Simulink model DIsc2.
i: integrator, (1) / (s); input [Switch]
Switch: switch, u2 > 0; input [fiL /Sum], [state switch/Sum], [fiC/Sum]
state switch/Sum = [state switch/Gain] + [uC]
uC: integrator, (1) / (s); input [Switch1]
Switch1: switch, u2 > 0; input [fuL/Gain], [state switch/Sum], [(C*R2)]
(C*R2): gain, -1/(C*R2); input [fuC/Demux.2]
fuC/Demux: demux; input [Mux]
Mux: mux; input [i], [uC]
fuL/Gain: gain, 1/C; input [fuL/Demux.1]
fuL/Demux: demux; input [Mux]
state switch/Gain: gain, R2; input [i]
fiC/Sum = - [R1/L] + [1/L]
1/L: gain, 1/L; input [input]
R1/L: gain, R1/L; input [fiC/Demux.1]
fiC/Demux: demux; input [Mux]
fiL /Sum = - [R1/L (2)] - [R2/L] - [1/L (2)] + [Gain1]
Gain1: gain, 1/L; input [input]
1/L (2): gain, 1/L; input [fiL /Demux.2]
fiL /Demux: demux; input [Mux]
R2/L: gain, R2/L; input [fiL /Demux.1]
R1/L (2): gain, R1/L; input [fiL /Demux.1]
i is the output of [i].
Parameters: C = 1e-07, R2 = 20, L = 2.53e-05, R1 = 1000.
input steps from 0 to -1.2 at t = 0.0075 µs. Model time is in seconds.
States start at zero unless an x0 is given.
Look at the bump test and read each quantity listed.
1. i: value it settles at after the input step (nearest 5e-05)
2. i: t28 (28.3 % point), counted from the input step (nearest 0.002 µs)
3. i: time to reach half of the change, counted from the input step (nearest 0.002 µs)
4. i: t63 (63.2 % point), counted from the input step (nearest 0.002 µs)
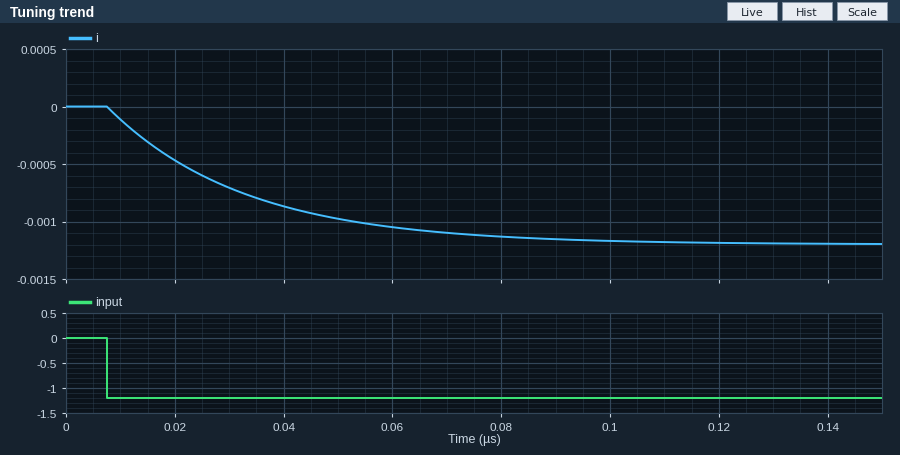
-0.00120
0.008 µs
0.018 µs
0.026 µs
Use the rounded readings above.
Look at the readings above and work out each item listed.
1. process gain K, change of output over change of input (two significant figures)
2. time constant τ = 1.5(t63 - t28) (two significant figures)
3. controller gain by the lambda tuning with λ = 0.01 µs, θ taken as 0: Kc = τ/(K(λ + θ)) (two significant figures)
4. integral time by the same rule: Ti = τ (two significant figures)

0.0010
0.027 µs
2700
0.027 µs
